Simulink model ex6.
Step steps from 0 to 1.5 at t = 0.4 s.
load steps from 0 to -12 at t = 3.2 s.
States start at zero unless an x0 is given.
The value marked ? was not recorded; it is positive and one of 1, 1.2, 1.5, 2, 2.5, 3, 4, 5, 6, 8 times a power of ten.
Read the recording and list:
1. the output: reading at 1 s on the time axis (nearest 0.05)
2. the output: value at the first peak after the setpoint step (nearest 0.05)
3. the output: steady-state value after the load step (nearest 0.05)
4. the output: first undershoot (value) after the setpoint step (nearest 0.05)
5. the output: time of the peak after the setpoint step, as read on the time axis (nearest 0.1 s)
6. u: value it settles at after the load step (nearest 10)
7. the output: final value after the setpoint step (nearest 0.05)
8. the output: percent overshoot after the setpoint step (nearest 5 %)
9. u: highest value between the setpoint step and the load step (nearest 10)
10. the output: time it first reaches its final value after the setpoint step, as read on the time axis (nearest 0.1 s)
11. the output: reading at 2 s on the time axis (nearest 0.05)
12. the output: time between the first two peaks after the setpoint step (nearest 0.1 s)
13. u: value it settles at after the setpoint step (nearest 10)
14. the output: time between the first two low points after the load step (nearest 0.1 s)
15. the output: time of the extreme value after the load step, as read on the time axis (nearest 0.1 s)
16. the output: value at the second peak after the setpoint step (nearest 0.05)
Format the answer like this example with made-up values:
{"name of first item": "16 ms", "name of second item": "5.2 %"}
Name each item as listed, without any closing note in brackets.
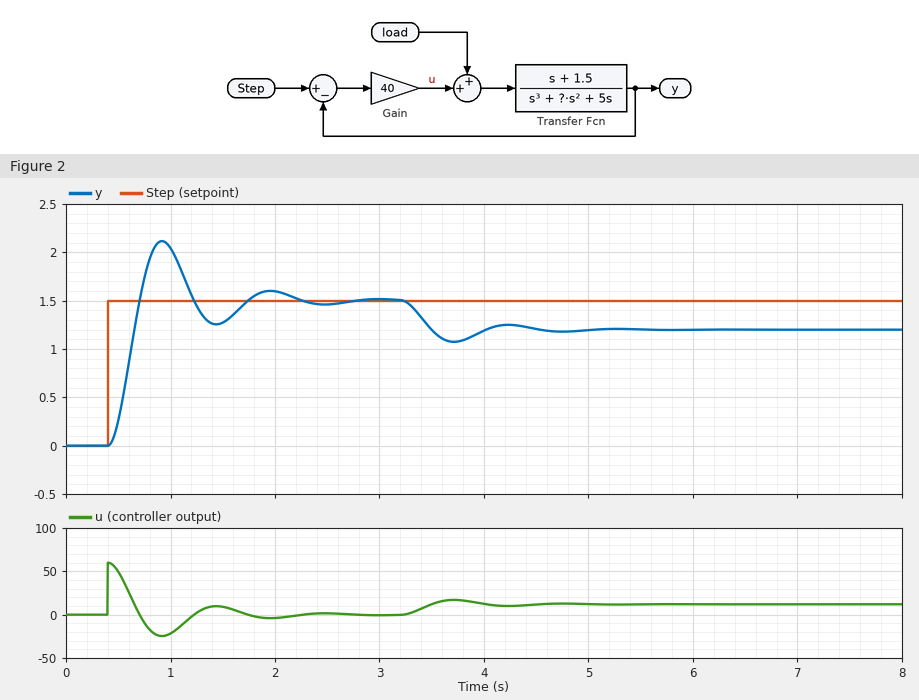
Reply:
{"the output: reading at 1 s on the time axis": "2.05", "the output: value at the first peak after the setpoint step": "2.10", "the output: steady-state value after the load step": "1.20", "the output: first undershoot (value) after the setpoint step": "1.25", "the output: time of the peak after the setpoint step, as read on the time axis": "0.9 s", "u: value it settles at after the load step": "10", "the output: final value after the setpoint step": "1.50", "the output: percent overshoot after the setpoint step": "40 %", "u: highest value between the setpoint step and the load step": "60", "the output: time it first reaches its final value after the setpoint step, as read on the time axis": "0.7 s", "the output: reading at 2 s on the time axis": "1.60", "the output: time between the first two peaks after the setpoint step": "1.0 s", "u: value it settles at after the setpoint step": "0", "the output: time between the first two low points after the load step": "1.0 s", "the output: time of the extreme value after the load step, as read on the time axis": "3.7 s", "the output: value at the second peak after the setpoint step": "1.60"}
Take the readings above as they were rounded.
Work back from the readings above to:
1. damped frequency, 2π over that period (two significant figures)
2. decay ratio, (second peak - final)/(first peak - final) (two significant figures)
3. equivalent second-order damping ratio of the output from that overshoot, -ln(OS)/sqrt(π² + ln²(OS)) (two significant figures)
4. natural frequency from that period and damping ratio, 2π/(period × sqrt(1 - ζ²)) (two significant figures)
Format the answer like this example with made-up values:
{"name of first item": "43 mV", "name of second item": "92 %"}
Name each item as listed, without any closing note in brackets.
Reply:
{"damped frequency, 2π over that period": "6.3 rad/s", "decay ratio, (second peak - final)/(first peak - final)": "0.17", "equivalent second-order damping ratio of the output from that overshoot, -ln(OS)/sqrt(π² + ln²(OS))": "0.28", "natural frequency from that period and damping ratio, 2π/(period × sqrt(1 - ζ²))": "6.5 rad/s"}
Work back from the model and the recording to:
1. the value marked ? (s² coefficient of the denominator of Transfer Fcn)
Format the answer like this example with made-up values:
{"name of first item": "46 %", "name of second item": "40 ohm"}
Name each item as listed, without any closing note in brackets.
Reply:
{"the value marked ?": "5"}
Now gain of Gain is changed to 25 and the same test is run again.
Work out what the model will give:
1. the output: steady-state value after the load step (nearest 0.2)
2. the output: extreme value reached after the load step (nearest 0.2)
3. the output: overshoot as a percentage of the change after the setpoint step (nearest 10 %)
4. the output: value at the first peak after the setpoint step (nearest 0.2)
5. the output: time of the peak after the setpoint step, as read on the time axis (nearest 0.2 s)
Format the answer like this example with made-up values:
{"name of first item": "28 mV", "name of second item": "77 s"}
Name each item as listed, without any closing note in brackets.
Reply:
{"the output: steady-state value after the load step": "1.0", "the output: extreme value reached after the load step": "0.8", "the output: overshoot as a percentage of the change after the setpoint step": "30 %", "the output: value at the first peak after the setpoint step": "2.0", "the output: time of the peak after the setpoint step, as read on the time axis": "1.0 s"}
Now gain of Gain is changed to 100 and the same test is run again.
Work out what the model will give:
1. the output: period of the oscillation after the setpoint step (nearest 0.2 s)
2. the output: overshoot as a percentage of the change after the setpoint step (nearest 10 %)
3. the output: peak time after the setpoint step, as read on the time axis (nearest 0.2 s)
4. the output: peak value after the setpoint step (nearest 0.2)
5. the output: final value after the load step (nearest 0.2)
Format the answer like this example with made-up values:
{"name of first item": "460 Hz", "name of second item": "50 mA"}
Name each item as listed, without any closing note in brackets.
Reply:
{"the output: period of the oscillation after the setpoint step": "0.6 s", "the output: overshoot as a percentage of the change after the setpoint step": "60 %", "the output: peak time after the setpoint step, as read on the time axis": "0.8 s", "the output: peak value after the setpoint step": "2.4", "the output: final value after the load step": "1.4"}
